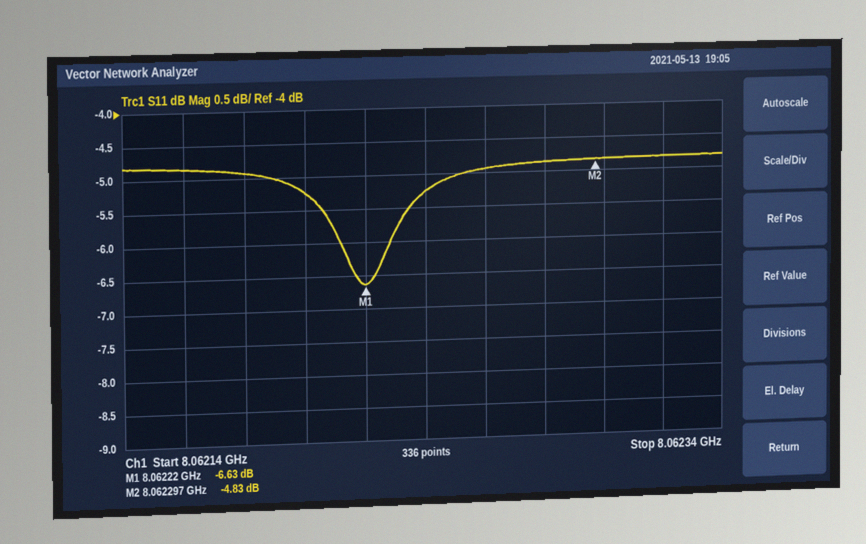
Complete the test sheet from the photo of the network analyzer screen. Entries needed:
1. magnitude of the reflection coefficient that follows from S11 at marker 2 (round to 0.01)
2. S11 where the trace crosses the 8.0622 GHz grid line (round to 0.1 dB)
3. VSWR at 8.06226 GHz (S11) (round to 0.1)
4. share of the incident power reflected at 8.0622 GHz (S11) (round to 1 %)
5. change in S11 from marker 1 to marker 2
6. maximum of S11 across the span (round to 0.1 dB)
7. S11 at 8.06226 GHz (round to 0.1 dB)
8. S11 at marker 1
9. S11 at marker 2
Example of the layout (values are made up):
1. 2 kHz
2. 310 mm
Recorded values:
1. 0.57
2. -5.2 dB
3. 3.6
4. 30 %
5. 1.80 dB
6. -4.8 dB
7. -4.9 dB
8. -6.63 dB
9. -4.83 dB
